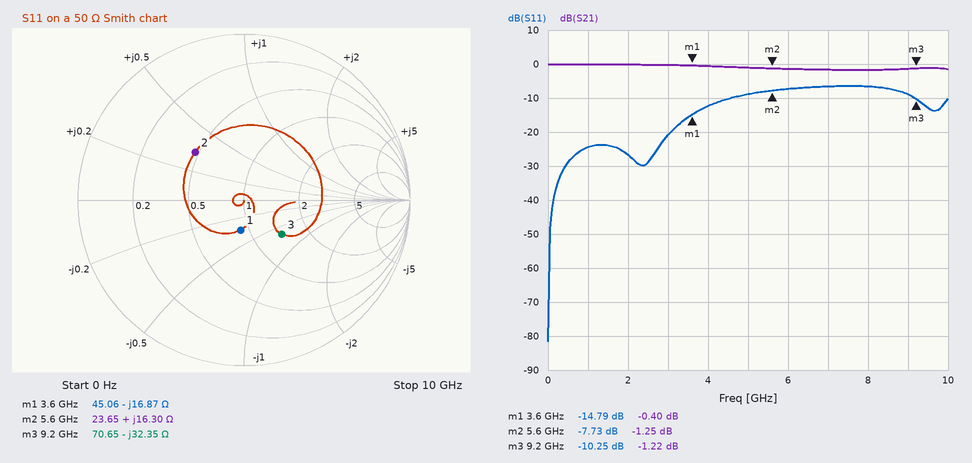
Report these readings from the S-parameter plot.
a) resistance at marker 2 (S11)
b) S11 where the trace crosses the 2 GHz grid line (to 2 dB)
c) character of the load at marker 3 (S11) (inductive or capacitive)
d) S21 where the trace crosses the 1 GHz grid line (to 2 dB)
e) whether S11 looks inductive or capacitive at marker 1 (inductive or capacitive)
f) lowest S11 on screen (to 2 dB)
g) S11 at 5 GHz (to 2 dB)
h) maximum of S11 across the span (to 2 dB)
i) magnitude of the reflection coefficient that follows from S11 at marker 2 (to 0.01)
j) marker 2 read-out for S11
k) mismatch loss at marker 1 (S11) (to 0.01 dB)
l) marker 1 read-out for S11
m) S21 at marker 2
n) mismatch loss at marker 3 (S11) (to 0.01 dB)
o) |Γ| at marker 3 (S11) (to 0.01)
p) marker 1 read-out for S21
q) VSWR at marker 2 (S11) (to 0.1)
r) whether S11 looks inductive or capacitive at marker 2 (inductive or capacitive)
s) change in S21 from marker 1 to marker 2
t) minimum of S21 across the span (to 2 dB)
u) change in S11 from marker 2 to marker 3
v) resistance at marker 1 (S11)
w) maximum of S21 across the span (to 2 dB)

23.65 Ω
-26 dB
capacitive
0 dB
capacitive
-82 dB
-8 dB
-6 dB
0.41
-7.73 dB
0.15 dB
-14.79 dB
-1.25 dB
0.43 dB
0.31
-0.40 dB
2.4
inductive
-0.85 dB
-2 dB
-2.52 dB
45.06 Ω
0 dB
